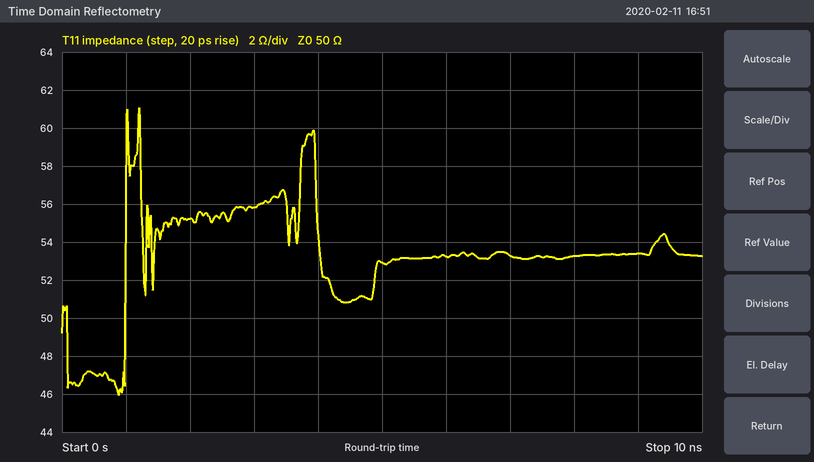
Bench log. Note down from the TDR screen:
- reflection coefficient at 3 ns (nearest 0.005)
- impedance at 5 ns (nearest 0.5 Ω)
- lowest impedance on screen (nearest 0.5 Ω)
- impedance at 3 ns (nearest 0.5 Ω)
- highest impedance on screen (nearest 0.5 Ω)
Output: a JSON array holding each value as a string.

["+0.055", "53.0 Ω", "46.0 Ω", "56.0 Ω", "61.0 Ω"]
